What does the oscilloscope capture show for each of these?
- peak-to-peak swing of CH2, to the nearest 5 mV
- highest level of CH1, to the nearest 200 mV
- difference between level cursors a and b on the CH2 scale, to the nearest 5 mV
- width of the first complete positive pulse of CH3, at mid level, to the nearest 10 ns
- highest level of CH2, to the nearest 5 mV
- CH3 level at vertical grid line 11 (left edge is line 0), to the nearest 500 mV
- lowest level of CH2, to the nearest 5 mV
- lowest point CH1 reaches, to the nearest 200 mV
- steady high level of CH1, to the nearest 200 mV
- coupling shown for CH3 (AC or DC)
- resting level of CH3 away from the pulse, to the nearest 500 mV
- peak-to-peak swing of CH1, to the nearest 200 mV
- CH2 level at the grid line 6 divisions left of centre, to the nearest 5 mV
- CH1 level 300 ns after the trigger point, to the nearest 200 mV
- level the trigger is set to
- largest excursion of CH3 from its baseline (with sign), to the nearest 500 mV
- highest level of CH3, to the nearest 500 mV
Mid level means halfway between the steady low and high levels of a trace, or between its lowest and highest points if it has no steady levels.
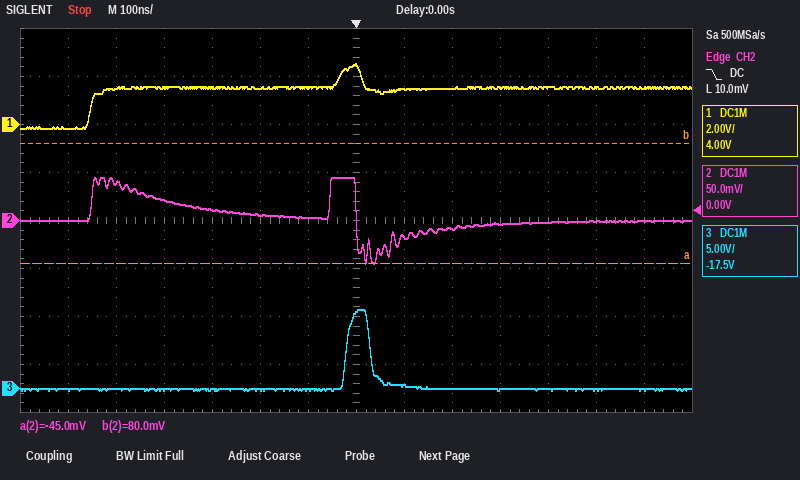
90 mV
2.6 V
125 mV
50 ns
45 mV
0.0 V
-45 mV
-200 mV
1.6 V
DC
0.0 V
2.8 V
0 mV
1.6 V
10.0 mV
+8.0 V
8.0 V
